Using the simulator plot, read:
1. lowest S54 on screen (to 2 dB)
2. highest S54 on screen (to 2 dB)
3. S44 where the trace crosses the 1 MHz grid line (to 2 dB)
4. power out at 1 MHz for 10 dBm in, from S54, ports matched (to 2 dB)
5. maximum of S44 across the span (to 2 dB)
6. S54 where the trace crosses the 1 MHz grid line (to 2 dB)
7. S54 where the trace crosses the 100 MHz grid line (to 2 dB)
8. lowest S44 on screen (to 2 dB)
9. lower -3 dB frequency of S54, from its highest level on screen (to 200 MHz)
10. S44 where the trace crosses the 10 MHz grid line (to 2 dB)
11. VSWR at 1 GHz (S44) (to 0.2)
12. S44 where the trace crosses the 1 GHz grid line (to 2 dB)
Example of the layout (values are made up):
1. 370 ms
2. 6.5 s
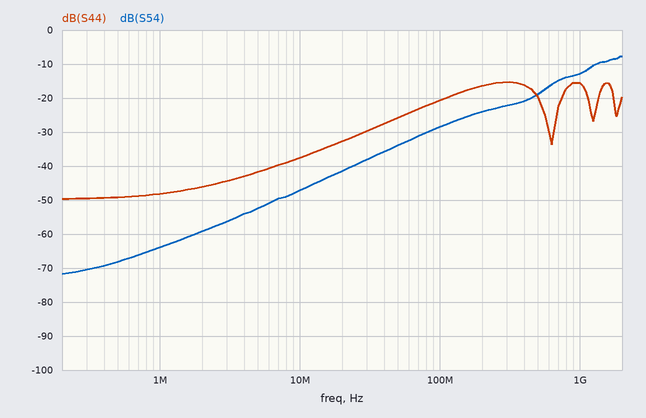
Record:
1. -72 dB
2. -8 dB
3. -48 dB
4. -54 dBm
5. -16 dB
6. -64 dB
7. -28 dB
8. -50 dB
9. 1.2 GHz
10. -38 dB
11. 1.4
12. -16 dB
